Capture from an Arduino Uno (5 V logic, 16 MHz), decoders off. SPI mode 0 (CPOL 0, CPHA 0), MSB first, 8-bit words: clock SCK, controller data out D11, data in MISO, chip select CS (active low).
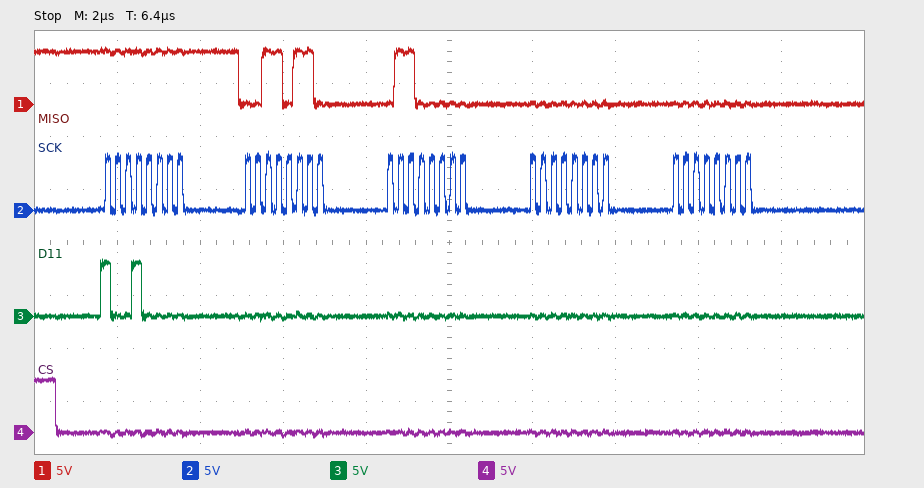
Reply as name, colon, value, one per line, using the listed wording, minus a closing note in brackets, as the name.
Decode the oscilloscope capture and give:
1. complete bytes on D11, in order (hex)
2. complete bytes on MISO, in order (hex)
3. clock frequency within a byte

complete bytes on D11, in order: 0x90 0x00 0x00 0x00 0x00
complete bytes on MISO, in order: 0xFF 0x36 0x60 0x00 0x00
clock frequency within a byte: 4 MHz
